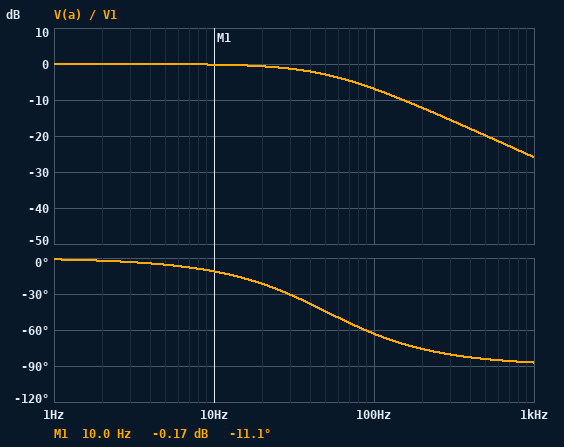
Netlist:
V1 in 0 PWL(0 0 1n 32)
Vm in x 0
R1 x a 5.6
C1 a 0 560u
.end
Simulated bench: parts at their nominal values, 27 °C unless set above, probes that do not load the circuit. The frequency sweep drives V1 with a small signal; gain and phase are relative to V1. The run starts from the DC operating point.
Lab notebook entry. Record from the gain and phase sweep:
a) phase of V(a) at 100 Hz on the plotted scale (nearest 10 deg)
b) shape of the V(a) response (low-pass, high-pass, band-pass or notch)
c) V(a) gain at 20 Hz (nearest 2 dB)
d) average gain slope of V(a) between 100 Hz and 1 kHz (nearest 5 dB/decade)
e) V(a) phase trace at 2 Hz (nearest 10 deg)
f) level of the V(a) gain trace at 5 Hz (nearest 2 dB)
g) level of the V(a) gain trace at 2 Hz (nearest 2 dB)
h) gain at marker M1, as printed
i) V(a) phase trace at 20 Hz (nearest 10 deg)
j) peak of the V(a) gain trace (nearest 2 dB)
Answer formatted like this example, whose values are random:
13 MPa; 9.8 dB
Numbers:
-60 deg; low-pass; 0 dB; -20 dB/decade; 0 deg; 0 dB; 0 dB; -0.17 dB; -20 deg; 0 dB
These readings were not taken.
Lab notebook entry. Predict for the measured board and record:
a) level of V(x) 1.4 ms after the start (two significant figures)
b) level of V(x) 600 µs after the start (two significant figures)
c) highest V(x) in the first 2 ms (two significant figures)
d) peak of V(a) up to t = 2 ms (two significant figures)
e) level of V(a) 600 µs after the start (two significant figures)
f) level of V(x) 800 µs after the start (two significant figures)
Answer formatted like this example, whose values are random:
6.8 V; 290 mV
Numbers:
32 V; 32 V; 32 V; 15 V; 5.6 V; 32 V
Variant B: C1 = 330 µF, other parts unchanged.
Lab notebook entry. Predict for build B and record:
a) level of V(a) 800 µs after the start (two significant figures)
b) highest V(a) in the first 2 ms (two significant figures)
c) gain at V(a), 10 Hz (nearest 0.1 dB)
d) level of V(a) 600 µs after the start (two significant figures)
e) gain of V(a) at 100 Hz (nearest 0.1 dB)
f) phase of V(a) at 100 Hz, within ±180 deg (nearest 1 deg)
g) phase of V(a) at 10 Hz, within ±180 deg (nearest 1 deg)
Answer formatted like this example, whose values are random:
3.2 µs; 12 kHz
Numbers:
11 V; 21 V; -0.1 dB; 8.9 V; -3.7 dB; -49 deg; -7 deg
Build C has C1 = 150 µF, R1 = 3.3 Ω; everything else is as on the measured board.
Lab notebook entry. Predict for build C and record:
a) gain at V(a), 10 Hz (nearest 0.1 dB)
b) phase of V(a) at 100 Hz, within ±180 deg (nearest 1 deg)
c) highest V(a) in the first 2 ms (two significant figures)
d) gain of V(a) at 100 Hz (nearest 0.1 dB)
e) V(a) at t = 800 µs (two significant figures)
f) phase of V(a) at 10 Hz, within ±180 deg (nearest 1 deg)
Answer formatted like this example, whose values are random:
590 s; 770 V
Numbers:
0 dB; -17 deg; 31 V; -0.4 dB; 26 V; -2 deg
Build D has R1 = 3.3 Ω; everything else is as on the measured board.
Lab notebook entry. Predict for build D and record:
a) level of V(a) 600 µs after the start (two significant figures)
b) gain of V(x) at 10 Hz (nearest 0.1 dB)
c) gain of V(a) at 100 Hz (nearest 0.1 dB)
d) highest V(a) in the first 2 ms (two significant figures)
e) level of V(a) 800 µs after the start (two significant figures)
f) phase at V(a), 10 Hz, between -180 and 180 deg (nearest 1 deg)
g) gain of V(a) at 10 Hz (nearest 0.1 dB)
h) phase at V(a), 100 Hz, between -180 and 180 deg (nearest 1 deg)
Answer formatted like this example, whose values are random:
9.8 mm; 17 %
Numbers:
8.9 V; 0 dB; -3.7 dB; 21 V; 11 V; -7 deg; -0.1 dB; -49 deg
